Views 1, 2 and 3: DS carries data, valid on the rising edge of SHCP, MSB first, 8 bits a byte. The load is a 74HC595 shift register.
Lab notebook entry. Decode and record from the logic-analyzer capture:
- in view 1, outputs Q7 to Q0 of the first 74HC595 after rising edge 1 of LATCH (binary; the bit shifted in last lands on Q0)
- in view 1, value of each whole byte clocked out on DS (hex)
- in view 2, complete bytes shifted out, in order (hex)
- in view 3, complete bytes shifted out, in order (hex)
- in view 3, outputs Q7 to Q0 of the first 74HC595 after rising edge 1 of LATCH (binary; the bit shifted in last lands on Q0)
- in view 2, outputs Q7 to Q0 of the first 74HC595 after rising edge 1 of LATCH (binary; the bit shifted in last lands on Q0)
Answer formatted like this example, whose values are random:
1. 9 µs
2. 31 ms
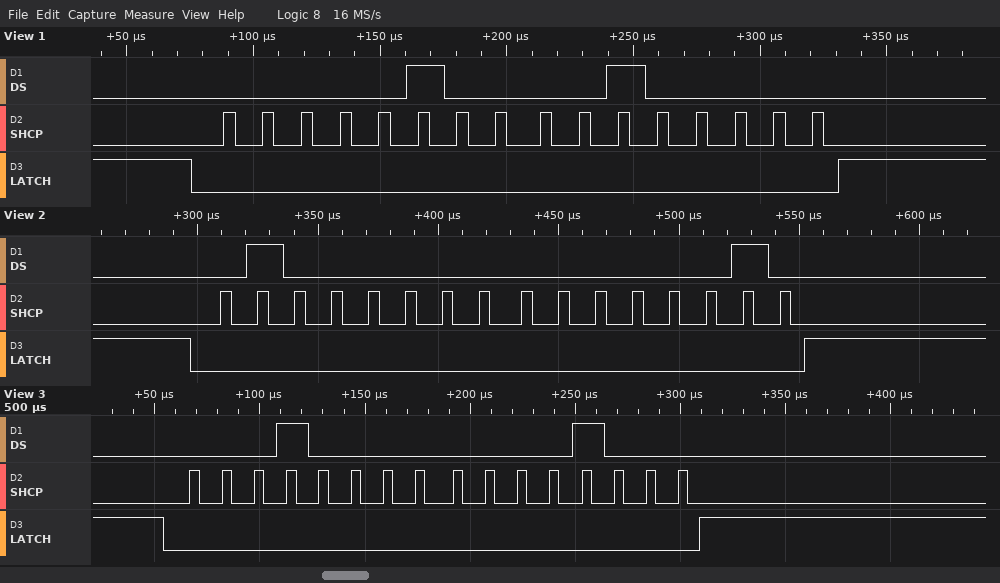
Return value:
1. 00100000
2. 04 20
3. 0x40 0x02
4. 10 08
5. 00001000
6. 00000010
